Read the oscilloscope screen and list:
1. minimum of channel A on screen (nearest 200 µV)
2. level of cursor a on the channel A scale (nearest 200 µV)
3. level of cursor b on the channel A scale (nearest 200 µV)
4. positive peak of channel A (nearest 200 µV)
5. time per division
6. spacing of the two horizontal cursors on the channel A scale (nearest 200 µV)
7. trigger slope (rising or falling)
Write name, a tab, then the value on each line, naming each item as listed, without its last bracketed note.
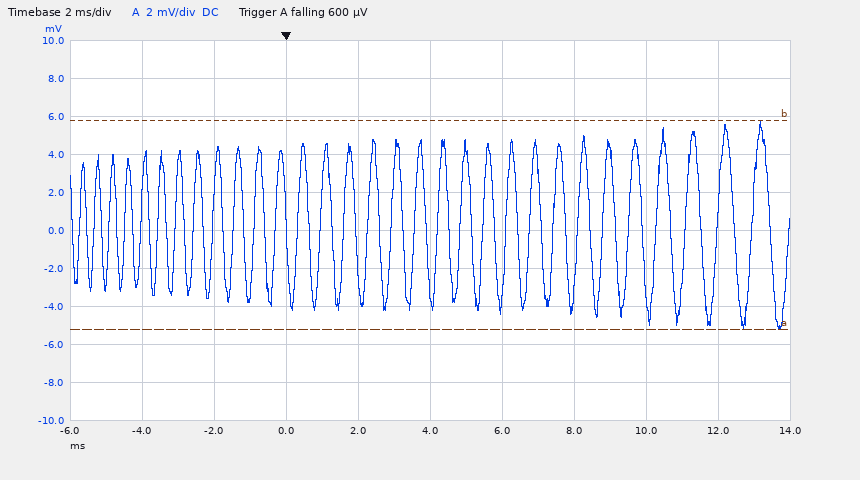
minimum of channel A on screen	-5.2 mV
level of cursor a on the channel A scale	-5.2 mV
level of cursor b on the channel A scale	5.8 mV
positive peak of channel A	5.8 mV
time per division	2 ms
spacing of the two horizontal cursors on the channel A scale	11.0 mV
trigger slope	falling
